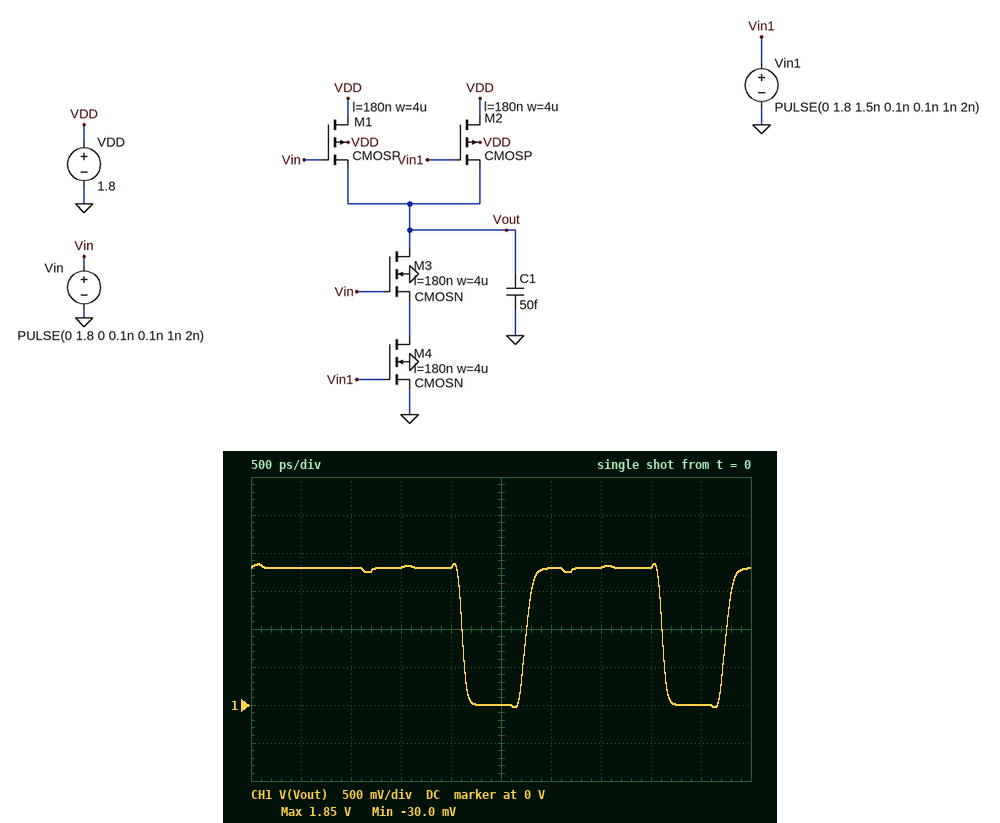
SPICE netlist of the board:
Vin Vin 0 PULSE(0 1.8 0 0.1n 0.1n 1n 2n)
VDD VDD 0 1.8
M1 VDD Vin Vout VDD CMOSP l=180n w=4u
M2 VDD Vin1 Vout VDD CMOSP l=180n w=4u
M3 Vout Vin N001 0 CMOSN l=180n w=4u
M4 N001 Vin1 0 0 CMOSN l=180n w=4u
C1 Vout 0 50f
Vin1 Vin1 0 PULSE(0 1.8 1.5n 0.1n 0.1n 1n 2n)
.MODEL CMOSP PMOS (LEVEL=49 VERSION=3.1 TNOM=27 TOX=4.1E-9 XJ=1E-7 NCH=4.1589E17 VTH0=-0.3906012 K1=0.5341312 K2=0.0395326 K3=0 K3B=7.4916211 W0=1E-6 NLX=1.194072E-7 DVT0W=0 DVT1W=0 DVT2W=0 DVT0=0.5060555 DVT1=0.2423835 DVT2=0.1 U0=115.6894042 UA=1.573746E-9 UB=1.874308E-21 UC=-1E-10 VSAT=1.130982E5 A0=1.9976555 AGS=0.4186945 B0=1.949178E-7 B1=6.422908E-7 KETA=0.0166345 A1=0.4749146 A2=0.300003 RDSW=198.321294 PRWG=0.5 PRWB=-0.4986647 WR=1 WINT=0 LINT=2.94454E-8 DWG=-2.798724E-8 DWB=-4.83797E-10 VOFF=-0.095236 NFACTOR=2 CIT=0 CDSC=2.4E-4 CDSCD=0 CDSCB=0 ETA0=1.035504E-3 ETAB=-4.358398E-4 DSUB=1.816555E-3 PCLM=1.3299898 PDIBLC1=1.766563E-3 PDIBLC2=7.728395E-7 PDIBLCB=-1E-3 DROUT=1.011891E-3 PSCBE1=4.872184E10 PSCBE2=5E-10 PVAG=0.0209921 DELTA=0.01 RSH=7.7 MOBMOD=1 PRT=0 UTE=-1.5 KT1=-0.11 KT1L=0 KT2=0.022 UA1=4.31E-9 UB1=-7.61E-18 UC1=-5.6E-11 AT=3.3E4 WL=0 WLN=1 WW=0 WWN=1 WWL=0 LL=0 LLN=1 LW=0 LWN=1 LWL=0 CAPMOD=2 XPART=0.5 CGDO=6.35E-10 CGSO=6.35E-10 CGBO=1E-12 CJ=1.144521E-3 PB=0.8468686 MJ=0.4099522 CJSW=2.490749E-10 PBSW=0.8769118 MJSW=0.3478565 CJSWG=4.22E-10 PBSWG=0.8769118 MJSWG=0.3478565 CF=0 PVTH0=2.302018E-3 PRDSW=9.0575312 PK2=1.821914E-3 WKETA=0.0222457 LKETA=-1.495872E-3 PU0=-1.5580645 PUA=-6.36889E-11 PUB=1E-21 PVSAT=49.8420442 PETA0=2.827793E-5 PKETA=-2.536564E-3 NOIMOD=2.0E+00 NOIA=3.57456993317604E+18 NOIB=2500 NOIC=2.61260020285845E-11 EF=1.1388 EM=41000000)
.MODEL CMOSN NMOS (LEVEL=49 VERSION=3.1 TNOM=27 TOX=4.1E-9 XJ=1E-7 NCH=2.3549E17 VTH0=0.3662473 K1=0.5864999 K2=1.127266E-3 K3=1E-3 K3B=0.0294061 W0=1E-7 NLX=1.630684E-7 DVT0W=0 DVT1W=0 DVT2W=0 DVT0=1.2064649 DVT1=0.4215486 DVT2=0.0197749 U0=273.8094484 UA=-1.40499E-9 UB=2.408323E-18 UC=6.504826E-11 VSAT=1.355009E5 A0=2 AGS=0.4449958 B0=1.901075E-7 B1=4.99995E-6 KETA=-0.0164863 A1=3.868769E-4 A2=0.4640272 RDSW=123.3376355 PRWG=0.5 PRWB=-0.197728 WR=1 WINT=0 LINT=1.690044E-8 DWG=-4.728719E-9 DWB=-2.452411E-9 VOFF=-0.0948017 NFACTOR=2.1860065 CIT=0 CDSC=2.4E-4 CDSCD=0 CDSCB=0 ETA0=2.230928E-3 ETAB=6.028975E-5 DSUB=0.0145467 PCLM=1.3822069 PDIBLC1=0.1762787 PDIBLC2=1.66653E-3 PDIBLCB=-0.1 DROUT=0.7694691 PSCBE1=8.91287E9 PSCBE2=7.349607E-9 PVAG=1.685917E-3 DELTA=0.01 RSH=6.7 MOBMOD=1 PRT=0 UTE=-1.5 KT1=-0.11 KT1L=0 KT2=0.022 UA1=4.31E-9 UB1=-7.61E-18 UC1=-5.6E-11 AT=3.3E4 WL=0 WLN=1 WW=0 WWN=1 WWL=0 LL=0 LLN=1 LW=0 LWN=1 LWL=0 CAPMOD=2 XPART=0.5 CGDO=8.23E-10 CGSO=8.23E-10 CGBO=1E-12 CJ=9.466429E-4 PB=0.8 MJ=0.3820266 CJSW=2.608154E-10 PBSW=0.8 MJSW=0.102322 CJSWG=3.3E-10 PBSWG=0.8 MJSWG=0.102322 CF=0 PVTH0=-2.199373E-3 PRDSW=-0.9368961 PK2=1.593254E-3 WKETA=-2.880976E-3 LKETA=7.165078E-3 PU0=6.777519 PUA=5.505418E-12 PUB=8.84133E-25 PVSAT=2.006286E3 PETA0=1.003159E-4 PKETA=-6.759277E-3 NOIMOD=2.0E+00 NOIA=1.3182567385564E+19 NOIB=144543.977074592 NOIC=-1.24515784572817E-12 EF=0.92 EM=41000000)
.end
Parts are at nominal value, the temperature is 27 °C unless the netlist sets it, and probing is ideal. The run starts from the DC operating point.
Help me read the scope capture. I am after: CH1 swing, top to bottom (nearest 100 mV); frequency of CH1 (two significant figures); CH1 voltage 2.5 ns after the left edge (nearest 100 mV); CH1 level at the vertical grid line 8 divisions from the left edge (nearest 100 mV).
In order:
1.9 V
500 MHz
0 V
1.8 V
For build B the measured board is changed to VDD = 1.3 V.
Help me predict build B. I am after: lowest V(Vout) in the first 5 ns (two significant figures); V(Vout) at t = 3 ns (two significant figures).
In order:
-56 mV
1.3 V
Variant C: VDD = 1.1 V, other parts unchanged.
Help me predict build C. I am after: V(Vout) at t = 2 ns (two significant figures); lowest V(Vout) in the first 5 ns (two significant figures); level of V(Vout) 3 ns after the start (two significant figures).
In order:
1.1 V
-73 mV
960 mV
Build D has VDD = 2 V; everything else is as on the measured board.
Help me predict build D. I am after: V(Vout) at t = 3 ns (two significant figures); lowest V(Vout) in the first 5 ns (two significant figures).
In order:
2.0 V
-26 mV
